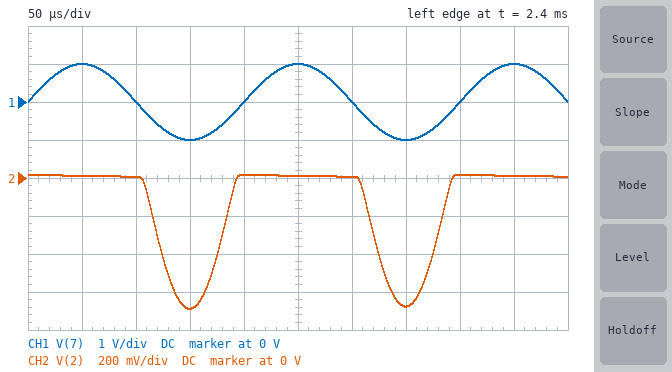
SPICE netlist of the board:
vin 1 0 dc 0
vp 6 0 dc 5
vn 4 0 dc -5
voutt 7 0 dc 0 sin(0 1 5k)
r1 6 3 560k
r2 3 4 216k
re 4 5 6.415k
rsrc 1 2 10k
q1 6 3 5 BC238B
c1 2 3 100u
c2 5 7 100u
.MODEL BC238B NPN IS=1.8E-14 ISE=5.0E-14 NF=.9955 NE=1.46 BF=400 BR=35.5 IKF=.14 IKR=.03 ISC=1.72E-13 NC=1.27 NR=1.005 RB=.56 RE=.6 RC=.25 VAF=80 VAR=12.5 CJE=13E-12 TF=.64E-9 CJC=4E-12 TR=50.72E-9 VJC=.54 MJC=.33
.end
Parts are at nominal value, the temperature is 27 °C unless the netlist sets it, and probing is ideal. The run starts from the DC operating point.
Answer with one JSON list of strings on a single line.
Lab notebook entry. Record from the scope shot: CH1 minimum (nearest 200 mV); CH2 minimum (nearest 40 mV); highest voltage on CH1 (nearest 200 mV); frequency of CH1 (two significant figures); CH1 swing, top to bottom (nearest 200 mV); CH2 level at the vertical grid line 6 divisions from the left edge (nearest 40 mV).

["-1.0 V", "-680 mV", "1.0 V", "5.0 kHz", "2.0 V", "0 V"]
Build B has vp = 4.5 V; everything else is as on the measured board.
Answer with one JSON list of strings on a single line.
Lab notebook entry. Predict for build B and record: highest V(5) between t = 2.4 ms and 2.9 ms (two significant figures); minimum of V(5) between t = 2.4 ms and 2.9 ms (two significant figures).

["-1.9 V", "-4.0 V"]
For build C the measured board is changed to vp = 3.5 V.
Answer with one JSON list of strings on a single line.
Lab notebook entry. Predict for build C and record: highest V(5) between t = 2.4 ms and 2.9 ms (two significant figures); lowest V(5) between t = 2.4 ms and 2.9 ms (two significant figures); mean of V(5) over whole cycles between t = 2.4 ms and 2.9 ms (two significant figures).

["-2.2 V", "-4.2 V", "-3.2 V"]
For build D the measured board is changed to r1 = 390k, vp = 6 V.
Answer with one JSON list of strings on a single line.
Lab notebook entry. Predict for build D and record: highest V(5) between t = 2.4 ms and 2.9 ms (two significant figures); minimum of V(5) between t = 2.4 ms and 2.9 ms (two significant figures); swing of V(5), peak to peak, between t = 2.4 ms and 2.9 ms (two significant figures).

["-740 mV", "-2.8 V", "2.0 V"]
